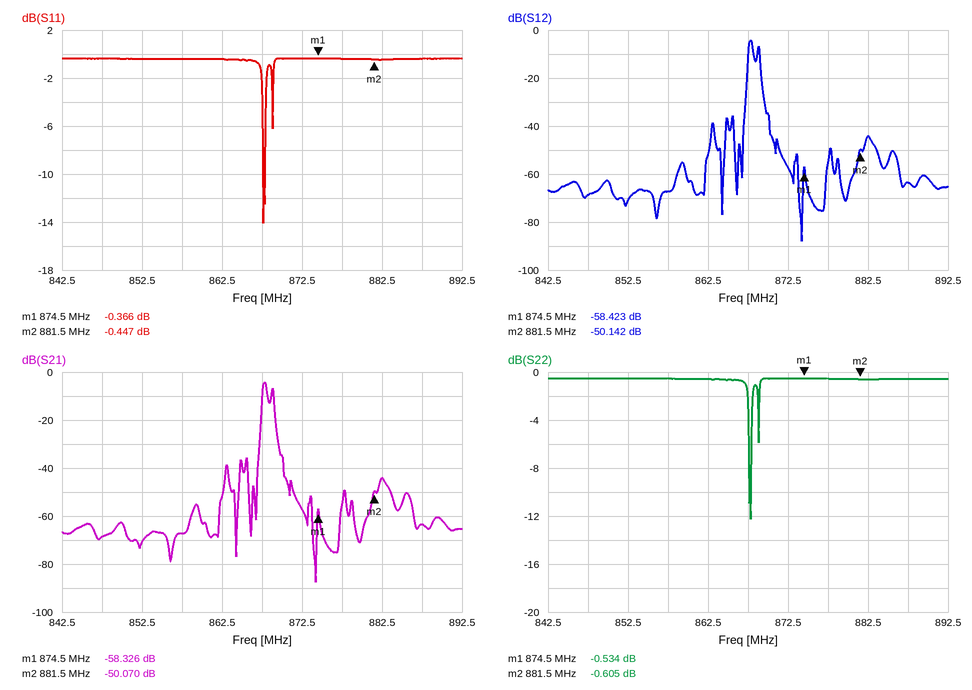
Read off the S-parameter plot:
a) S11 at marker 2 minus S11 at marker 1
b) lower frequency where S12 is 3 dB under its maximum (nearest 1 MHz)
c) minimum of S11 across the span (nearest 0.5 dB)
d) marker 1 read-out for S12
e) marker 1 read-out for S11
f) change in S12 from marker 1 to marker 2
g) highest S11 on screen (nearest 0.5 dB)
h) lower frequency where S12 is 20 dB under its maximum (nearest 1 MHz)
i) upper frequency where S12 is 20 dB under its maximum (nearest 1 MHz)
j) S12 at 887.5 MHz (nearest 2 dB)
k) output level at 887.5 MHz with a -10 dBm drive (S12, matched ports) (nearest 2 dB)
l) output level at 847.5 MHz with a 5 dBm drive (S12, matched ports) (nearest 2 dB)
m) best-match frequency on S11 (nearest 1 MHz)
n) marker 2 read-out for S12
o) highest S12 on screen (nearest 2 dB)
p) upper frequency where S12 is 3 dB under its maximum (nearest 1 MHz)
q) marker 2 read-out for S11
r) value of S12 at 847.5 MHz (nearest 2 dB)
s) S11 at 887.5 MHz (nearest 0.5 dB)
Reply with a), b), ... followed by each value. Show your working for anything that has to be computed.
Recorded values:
a) -0.447 − (-0.366) = -0.081 dB
b) 868 MHz
c) -14.0 dB
d) -58.423 dB
e) -0.366 dB
f) -50.142 − (-58.423) = 8.281 dB
g) -0.5 dB
h) 867 MHz
i) 869 MHz
j) -64 dB
k) -10 dBm + (-64 dB) = -74 dBm
l) 5 dBm + (-68 dB) = -64 dBm
m) 868 MHz
n) -50.142 dB
o) -4 dB
p) 868 MHz
q) -0.447 dB
r) -68 dB
s) -0.5 dB
